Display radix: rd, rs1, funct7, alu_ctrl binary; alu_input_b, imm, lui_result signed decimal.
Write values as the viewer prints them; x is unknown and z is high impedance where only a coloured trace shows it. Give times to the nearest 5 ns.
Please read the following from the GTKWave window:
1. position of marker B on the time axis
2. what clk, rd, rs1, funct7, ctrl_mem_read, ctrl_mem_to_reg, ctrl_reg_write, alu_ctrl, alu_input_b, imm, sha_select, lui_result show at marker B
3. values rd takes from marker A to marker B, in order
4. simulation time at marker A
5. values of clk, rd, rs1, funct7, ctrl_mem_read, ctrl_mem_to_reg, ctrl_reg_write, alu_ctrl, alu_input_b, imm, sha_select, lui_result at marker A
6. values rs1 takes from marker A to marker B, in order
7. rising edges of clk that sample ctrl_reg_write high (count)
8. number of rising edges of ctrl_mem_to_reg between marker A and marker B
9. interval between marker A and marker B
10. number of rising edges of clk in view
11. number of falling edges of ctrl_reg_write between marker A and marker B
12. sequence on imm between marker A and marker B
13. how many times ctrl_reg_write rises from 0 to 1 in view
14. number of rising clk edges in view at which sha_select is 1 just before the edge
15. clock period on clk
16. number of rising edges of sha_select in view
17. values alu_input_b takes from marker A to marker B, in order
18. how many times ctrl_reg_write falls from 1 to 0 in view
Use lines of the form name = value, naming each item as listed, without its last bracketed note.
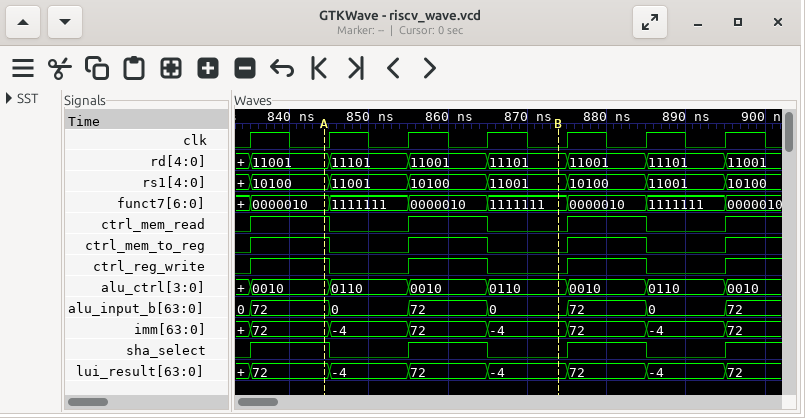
position of marker B on the time axis = 875 ns
what clk, rd, rs1, funct7, ctrl_mem_read, ctrl_mem_to_reg, ctrl_reg_write, alu_ctrl, alu_input_b, imm, sha_select, lui_result show at marker B = clk=0, rd=11101, rs1=11001, funct7=1111111, ctrl_mem_read=0, ctrl_mem_to_reg=0, ctrl_reg_write=0, alu_ctrl=0110, alu_input_b=0, imm=-4, sha_select=0, lui_result=-4
values rd takes from marker A to marker B, in order = 11001, 11101, 11001, 11101
simulation time at marker A = 845 ns
values of clk, rd, rs1, funct7, ctrl_mem_read, ctrl_mem_to_reg, ctrl_reg_write, alu_ctrl, alu_input_b, imm, sha_select, lui_result at marker A = clk=0, rd=11001, rs1=10100, funct7=0000010, ctrl_mem_read=1, ctrl_mem_to_reg=1, ctrl_reg_write=1, alu_ctrl=0010, alu_input_b=72, imm=72, sha_select=1, lui_result=72
values rs1 takes from marker A to marker B, in order = 10100, 11001, 10100, 11001
rising edges of clk that sample ctrl_reg_write high = 3
number of rising edges of ctrl_mem_to_reg between marker A and marker B = 1
interval between marker A and marker B = 30 ns
number of rising edges of clk in view = 7
number of falling edges of ctrl_reg_write between marker A and marker B = 2
sequence on imm between marker A and marker B = 72, -4, 72, -4
how many times ctrl_reg_write rises from 0 to 1 in view = 4
number of rising clk edges in view at which sha_select is 1 just before the edge = 3
clock period on clk = 10 ns
number of rising edges of sha_select in view = 4
values alu_input_b takes from marker A to marker B, in order = 72, 0, 72, 0
how many times ctrl_reg_write falls from 1 to 0 in view = 3
